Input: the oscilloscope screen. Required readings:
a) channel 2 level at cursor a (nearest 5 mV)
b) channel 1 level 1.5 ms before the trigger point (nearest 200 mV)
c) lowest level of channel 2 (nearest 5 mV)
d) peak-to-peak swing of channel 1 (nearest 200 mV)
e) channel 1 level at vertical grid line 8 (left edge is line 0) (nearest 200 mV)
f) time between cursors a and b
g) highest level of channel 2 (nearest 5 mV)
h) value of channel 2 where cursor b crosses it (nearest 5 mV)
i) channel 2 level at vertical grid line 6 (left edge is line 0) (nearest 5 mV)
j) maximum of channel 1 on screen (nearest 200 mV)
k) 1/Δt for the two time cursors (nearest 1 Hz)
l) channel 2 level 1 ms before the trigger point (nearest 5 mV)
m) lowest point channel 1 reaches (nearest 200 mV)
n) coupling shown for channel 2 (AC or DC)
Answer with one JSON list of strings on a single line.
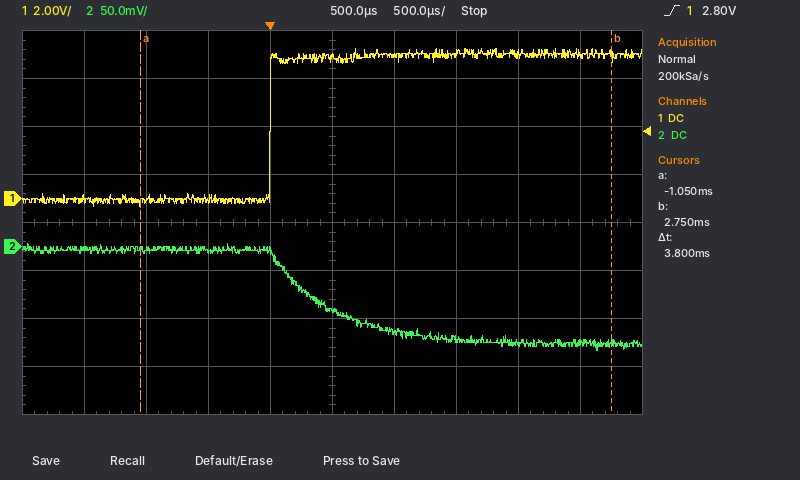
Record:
["-5 mV", "0.0 V", "-110 mV", "6.6 V", "6.0 V", "3.8 ms", "5 mV", "-100 mV", "-90 mV", "6.2 V", "263 Hz", "-5 mV", "-400 mV", "DC"]
